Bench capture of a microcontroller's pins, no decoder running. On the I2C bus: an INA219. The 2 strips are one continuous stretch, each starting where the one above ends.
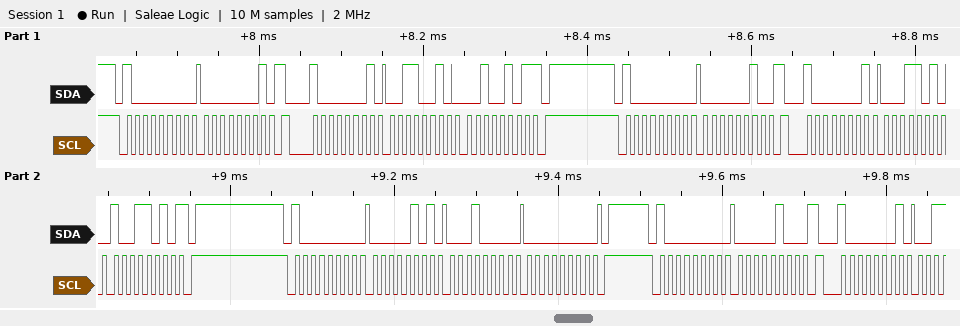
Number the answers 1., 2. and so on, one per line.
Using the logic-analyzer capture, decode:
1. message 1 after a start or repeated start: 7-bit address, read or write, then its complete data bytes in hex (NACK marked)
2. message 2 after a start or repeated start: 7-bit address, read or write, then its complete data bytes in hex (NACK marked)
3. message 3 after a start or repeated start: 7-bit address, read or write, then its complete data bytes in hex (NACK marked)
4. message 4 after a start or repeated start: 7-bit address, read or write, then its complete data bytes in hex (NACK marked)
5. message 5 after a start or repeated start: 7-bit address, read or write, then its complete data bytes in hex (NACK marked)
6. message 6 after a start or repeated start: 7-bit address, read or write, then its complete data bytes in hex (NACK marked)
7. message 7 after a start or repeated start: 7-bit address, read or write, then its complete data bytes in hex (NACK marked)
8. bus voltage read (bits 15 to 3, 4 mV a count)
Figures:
1. 0x40 write: 01
2. 0x40 read: 32 25 NACK
3. 0x40 write: 02
4. 0x40 read: 1A 9A NACK
5. 0x40 write: 05 10 00
6. 0x40 write: 04
7. 0x40 read
8. 3.404 V
